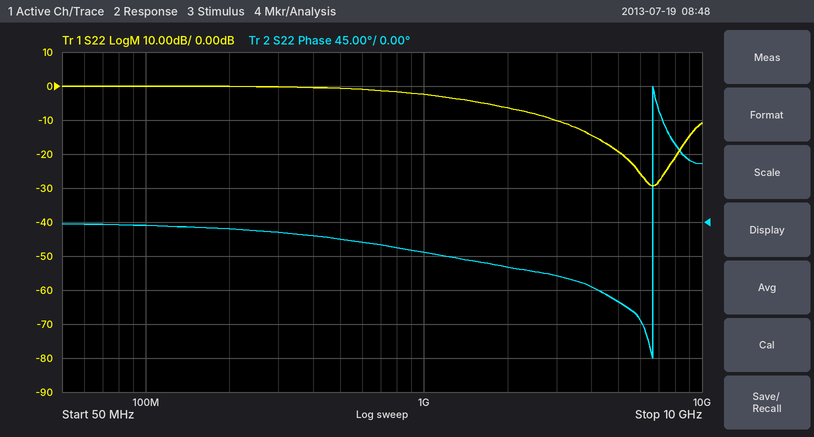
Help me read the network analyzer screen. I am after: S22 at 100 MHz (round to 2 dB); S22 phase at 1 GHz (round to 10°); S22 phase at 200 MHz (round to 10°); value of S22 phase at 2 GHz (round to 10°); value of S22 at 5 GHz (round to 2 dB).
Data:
0 dB
-40°
-10°
-60°
-20 dB
